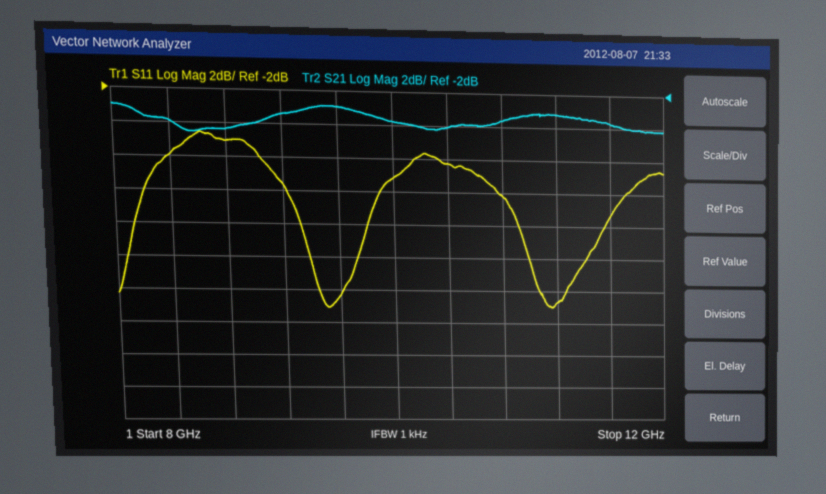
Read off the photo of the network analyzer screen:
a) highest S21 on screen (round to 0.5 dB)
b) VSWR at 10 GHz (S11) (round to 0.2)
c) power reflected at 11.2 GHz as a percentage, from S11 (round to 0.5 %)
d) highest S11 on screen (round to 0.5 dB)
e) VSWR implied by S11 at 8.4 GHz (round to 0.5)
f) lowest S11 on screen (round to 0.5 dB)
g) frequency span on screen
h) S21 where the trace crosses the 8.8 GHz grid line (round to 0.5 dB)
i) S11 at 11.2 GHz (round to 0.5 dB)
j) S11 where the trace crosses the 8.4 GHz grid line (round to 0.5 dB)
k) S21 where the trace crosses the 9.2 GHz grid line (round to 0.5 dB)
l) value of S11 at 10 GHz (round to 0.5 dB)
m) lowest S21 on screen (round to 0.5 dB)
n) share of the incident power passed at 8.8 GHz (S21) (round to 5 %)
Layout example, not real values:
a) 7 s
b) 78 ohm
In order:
a) -3.0 dB
b) 2.6
c) 3.5 %
d) -4.5 dB
e) 3.0
f) -15.0 dB
g) 4 GHz
h) -4.5 dB
i) -14.5 dB
j) -6.0 dB
k) -3.5 dB
l) -7.0 dB
m) -4.5 dB
n) 35 %
